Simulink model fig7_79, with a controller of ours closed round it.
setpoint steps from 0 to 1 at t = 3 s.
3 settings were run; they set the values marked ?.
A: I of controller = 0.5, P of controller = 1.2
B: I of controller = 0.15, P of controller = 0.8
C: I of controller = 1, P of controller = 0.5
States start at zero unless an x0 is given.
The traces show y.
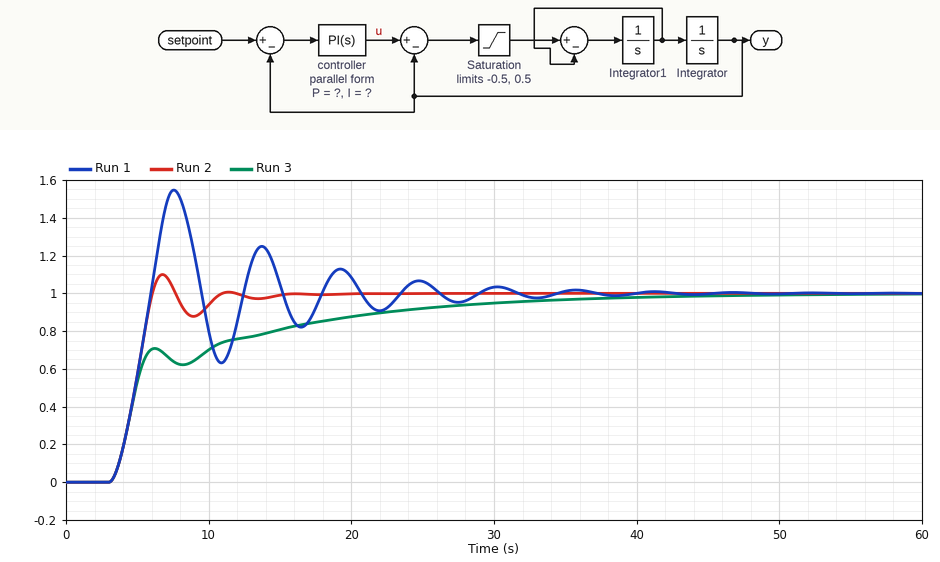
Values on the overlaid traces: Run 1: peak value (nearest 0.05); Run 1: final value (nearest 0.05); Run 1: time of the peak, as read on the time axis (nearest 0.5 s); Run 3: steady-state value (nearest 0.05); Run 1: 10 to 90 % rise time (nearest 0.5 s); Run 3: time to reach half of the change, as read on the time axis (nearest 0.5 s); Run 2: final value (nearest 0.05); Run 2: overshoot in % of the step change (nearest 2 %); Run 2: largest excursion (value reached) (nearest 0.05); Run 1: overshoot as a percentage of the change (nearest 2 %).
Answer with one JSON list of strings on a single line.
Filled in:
["1.55", "1.00", "7.5 s", "1.00", "2.0 s", "5.0 s", "1.00", "10 %", "1.10", "54 %"]
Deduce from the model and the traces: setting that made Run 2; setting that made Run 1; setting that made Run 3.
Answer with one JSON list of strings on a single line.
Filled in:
["A", "C", "B"]
